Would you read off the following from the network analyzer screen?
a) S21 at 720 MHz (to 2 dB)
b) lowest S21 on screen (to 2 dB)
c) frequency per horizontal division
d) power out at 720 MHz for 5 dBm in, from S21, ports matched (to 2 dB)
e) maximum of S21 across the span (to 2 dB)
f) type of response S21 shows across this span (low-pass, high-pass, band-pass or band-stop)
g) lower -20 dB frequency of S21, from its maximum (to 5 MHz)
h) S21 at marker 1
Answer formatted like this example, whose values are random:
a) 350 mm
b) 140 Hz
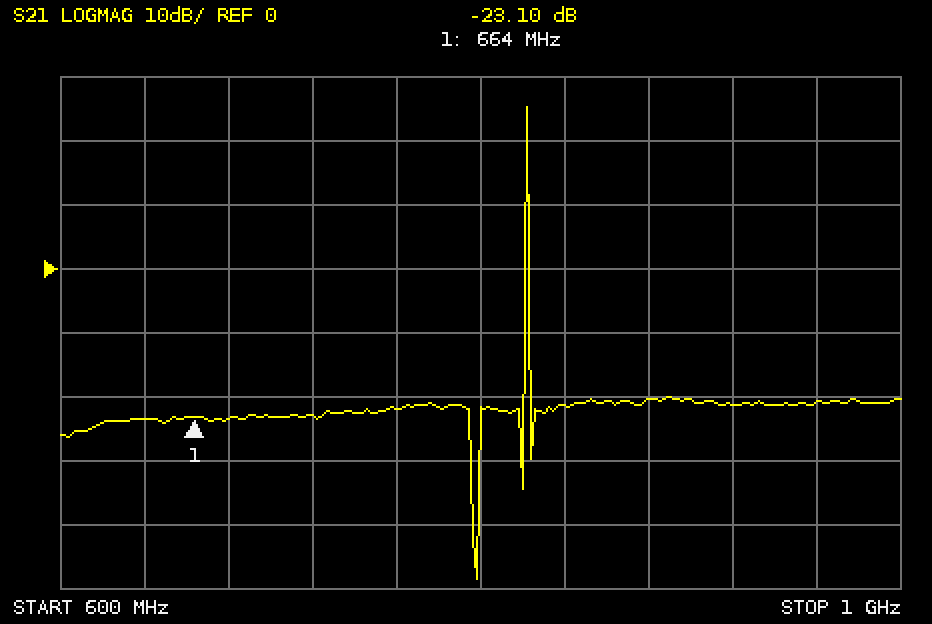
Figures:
a) -22 dB
b) -48 dB
c) 40 MHz
d) -18 dBm
e) 26 dB
f) band-pass
g) 820 MHz
h) -23.10 dB
